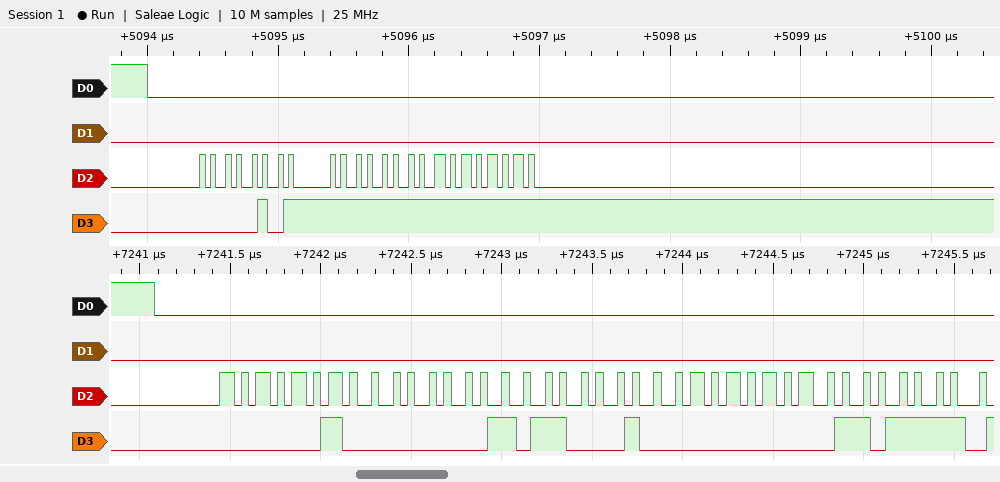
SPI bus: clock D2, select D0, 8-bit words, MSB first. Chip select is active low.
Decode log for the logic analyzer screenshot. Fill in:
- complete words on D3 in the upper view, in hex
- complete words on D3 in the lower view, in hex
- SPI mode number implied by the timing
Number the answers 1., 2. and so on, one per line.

1. 05, FF, FF
2. 02, 01, 62, 00, 6F
3. 0
